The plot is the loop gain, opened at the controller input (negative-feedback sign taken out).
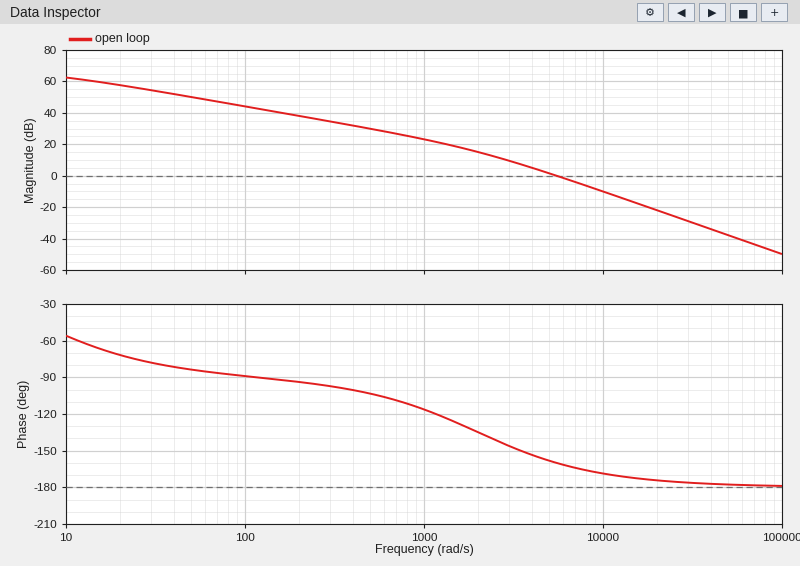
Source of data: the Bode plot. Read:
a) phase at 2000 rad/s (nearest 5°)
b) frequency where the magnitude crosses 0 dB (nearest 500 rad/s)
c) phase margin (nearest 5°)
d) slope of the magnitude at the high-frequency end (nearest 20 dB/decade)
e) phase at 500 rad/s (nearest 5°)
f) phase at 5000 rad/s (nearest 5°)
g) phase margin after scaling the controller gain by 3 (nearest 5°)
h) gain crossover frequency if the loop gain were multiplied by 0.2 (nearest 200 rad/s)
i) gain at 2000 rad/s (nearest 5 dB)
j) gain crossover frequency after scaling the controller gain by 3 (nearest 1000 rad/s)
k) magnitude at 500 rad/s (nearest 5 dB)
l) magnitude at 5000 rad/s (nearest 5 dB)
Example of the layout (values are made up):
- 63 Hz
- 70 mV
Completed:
- -135°
- 5500 rad/s
- 20°
- -40 dB/decade
- -105°
- -160°
- 10°
- 2200 rad/s
- 15 dB
- 10000 rad/s
- 30 dB
- 0 dB
